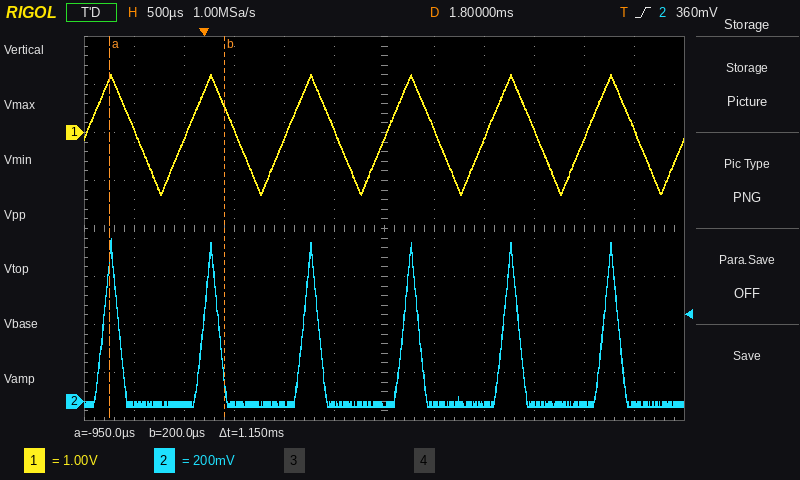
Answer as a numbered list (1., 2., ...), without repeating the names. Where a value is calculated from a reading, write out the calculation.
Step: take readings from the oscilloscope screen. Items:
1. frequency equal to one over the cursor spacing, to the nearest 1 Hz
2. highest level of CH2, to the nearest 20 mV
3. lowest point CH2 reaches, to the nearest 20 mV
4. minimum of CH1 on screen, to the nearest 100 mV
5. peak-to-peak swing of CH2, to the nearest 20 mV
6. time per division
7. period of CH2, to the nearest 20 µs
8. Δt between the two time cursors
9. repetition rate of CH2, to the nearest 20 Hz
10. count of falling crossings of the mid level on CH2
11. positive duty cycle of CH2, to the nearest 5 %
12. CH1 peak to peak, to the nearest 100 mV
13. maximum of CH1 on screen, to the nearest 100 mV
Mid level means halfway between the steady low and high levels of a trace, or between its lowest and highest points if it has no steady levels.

1. 1 / 1.15 ms ≈ 870 Hz
2. 680 mV
3. -20 mV
4. -1.3 V
5. 680 mV − (-20 mV) = 700 mV
6. 500 µs
7. 1.00 ms
8. 1.15 ms
9. 1 / 1.00 ms ≈ 1.00 kHz
10. 6
11. 15 %
12. 1.2 V − (-1.3 V) = 2.5 V
13. 1.2 V
